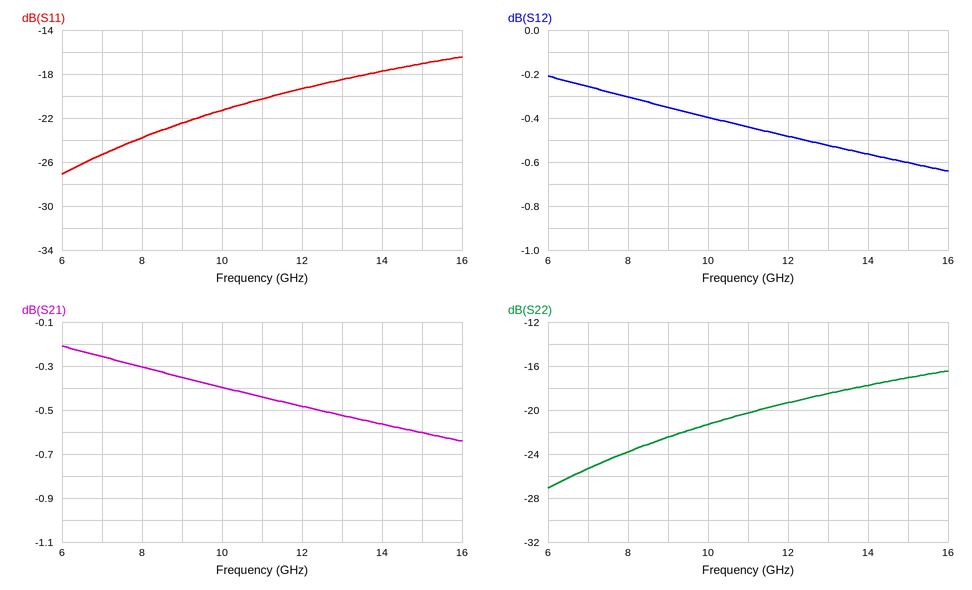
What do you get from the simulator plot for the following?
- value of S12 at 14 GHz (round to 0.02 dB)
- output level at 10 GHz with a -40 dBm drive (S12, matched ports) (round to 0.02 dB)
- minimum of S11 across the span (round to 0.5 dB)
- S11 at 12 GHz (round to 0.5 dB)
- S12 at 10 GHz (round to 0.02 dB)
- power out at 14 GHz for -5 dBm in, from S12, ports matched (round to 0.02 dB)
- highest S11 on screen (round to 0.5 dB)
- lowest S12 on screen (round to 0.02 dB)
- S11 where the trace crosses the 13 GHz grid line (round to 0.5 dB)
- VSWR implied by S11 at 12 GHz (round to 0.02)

-0.56 dB
-40.40 dBm
-27.0 dB
-19.5 dB
-0.40 dB
-5.56 dBm
-16.5 dB
-0.64 dB
-18.5 dB
1.24
